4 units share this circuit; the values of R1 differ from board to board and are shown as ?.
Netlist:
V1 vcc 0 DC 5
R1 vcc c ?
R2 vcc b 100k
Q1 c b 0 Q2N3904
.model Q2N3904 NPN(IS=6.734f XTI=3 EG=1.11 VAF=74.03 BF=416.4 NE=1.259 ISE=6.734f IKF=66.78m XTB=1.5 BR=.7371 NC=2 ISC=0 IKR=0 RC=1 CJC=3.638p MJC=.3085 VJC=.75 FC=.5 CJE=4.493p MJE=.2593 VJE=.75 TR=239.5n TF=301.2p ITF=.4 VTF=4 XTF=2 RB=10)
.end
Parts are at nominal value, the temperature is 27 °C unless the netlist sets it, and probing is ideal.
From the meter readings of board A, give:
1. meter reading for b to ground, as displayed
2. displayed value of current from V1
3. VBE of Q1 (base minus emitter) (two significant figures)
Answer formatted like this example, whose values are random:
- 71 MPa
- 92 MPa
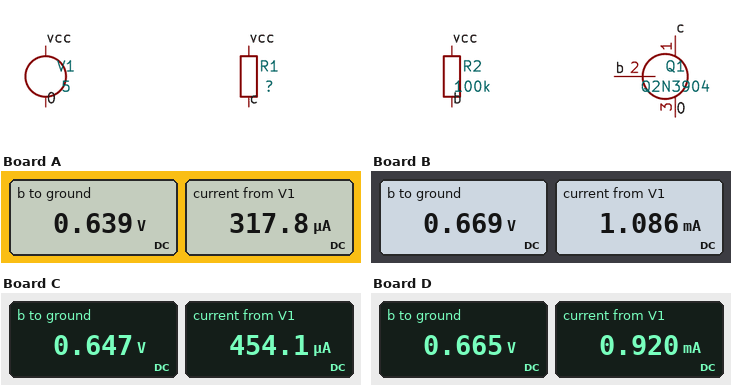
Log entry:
- 0.639 V
- 317.8 µA
- 640 mV
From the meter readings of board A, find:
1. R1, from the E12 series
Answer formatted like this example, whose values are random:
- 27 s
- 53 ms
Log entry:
- 18 kΩ
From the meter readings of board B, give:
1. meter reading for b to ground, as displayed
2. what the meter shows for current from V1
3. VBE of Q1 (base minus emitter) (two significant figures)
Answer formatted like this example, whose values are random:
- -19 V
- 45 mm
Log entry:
- 0.669 V
- 1.086 mA
- 670 mV
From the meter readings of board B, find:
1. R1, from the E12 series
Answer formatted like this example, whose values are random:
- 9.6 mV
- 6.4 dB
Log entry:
- 4.7 kΩ
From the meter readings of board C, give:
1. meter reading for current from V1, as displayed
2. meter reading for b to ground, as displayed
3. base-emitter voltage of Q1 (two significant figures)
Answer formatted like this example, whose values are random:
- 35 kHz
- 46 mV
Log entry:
- 454.1 µA
- 0.647 V
- 650 mV
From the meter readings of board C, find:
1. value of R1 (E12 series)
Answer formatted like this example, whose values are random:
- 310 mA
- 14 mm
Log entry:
- 12 kΩ
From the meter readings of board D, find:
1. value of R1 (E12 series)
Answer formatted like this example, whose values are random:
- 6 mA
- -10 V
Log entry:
- 5.6 kΩ
